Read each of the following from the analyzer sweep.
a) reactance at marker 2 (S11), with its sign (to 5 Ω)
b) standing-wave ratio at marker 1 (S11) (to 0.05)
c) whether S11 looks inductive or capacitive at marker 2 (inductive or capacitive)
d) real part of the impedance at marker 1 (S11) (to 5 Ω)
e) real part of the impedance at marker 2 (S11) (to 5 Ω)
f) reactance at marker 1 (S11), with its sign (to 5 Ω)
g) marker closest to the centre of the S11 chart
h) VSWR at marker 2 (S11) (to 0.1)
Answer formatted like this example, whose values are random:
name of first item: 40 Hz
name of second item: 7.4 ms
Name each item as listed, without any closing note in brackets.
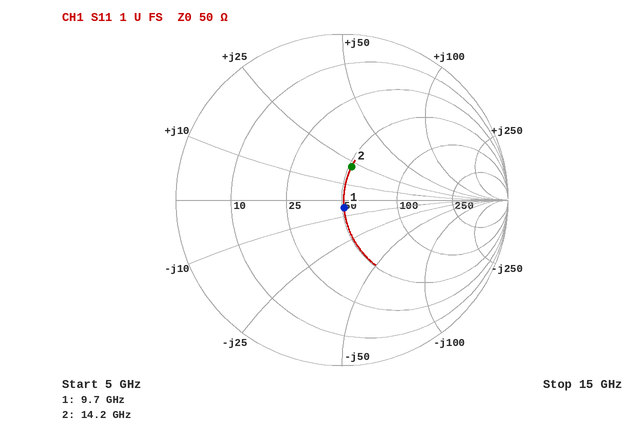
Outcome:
reactance at marker 2 (S11), with its sign: +20 Ω
standing-wave ratio at marker 1 (S11): 1.10
whether S11 looks inductive or capacitive at marker 2: inductive
real part of the impedance at marker 1 (S11): 50 Ω
real part of the impedance at marker 2 (S11): 50 Ω
reactance at marker 1 (S11), with its sign: -5 Ω
marker closest to the centre of the S11 chart: marker 1
VSWR at marker 2 (S11): 1.5
